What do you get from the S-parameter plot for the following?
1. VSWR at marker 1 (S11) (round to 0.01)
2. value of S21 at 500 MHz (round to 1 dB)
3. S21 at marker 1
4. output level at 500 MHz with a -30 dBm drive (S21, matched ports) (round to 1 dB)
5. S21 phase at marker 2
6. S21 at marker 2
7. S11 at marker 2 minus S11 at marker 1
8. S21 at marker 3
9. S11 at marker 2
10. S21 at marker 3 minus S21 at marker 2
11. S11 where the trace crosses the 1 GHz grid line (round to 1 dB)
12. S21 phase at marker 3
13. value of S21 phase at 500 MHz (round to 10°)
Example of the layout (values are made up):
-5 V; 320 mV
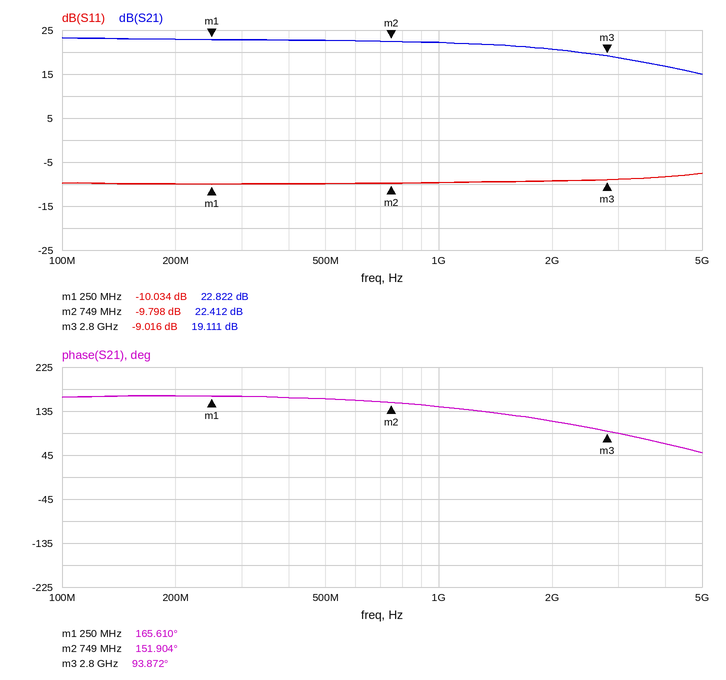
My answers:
1.92; 23 dB; 22.822 dB; -7 dBm; 151.904°; 22.412 dB; 0.236 dB; 19.111 dB; -9.798 dB; -3.301 dB; -10 dB; 93.872°; 160°
